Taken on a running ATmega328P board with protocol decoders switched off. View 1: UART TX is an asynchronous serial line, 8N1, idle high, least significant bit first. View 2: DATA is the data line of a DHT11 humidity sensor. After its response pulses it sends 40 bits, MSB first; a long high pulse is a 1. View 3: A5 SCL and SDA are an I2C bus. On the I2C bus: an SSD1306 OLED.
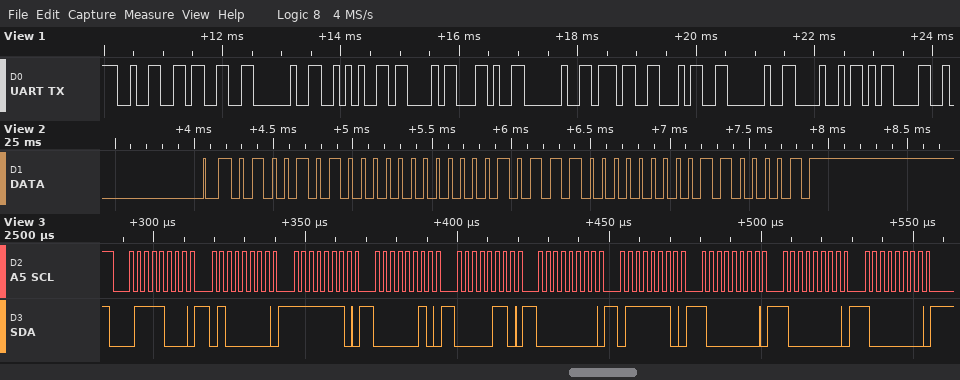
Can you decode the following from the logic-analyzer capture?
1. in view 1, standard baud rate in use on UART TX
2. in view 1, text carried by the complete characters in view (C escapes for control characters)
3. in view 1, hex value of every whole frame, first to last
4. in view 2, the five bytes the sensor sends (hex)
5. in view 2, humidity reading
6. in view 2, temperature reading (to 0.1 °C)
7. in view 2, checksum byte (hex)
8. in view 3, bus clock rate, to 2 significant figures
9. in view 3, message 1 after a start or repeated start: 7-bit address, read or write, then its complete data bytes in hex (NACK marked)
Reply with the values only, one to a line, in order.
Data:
9600 baud
"23 *C, 74 H\r"
32 33 20 2A 43 2C 20 37 34 20 48 0D
4A 00 17 00 61
74 %
23.0 °C
0x61
400 kHz
0x3C write: 40 FE 02 06 00 7E 80 80 80
